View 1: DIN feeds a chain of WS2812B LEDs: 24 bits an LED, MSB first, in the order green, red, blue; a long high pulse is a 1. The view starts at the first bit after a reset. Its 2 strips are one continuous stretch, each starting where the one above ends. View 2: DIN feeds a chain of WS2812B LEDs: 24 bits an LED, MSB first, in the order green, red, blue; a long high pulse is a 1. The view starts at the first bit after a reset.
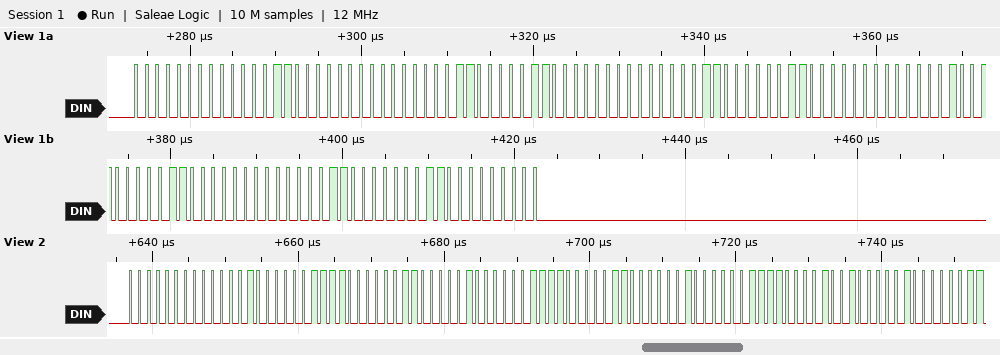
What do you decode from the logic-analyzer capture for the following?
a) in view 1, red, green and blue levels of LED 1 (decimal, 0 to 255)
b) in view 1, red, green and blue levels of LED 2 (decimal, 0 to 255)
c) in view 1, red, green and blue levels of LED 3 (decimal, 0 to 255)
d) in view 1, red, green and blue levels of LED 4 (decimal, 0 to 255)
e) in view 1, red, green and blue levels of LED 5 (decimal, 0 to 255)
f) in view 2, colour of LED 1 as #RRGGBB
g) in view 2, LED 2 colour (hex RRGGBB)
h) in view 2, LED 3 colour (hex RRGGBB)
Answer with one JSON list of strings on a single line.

["6, 0, 0", "6, 3, 0", "6, 6, 0", "6, 9, 0", "6, 12, 0", "#04000F", "#04030F", "#04060F"]
